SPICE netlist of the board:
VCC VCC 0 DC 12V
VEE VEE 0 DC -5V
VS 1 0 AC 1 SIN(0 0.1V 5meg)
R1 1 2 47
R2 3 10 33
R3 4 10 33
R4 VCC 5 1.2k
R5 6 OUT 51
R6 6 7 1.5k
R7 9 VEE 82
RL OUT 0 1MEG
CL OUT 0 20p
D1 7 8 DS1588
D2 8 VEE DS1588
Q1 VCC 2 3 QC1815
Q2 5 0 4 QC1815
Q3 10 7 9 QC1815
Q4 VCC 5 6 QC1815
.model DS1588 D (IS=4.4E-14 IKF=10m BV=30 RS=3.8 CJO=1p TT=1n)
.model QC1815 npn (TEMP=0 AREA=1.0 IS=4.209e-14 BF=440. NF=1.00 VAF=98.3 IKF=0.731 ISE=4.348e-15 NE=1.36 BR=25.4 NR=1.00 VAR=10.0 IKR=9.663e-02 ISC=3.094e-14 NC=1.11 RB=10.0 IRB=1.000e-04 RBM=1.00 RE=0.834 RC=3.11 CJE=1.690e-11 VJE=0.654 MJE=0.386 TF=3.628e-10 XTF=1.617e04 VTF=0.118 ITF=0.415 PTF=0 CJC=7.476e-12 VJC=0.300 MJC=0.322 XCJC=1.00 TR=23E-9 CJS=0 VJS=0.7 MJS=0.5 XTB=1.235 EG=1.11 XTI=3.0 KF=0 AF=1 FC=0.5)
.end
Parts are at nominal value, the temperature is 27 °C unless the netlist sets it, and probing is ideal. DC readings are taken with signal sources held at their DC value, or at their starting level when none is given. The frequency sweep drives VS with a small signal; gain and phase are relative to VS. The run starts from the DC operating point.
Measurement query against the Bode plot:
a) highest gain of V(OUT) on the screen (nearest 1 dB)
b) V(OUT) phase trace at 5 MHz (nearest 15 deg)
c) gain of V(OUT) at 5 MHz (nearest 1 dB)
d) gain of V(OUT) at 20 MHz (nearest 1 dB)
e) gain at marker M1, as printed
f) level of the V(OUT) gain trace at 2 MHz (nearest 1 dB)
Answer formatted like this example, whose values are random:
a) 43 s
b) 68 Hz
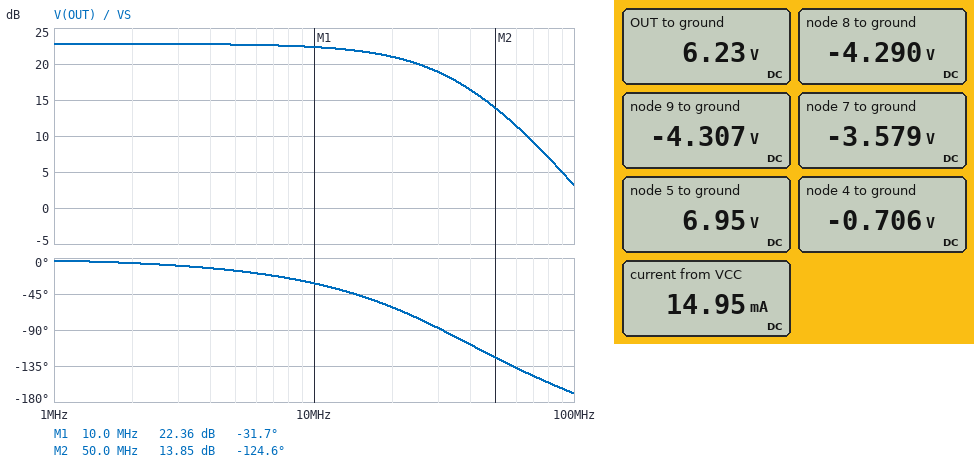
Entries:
a) 23 dB
b) -15 deg
c) 23 dB
d) 21 dB
e) 22.36 dB
f) 23 dB
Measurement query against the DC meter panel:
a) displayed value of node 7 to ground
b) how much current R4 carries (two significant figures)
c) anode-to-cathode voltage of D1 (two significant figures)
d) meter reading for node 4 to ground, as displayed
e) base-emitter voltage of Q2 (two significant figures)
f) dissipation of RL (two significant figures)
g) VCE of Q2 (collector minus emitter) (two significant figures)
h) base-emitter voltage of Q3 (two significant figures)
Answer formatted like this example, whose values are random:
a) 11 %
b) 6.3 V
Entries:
a) -3.579 V
b) 4.2 mA
c) 710 mV
d) -0.706 V
e) 710 mV
f) 39 µW
g) 7.7 V
h) 730 mV
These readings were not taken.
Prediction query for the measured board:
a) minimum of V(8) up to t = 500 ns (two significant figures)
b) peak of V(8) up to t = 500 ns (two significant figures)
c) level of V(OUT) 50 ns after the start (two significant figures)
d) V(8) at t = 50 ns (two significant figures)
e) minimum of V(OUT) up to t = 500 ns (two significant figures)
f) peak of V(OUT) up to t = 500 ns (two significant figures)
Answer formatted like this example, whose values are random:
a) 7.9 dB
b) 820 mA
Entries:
a) -4.3 V
b) -4.3 V
c) 7.5 V
d) -4.3 V
e) 4.9 V
f) 7.6 V
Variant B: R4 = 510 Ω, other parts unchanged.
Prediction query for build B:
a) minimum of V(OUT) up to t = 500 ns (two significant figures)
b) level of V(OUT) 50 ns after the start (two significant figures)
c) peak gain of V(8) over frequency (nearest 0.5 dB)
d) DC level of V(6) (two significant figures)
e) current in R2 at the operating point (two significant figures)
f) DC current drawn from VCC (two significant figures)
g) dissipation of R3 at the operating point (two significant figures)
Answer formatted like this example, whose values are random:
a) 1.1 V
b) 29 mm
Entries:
a) 8.4 V
b) 9.6 V
c) -29.5 dB
d) 9.0 V
e) 4.4 mA
f) 17 mA
g) 640 µW
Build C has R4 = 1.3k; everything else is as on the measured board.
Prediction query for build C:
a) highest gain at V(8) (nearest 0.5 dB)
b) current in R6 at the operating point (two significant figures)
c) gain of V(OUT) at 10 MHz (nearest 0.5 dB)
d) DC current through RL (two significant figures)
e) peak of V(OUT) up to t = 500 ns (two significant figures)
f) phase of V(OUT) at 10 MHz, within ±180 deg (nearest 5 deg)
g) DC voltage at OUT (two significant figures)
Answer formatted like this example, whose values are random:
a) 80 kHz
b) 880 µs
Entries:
a) -20.5 dB
b) 6.3 mA
c) 23.0 dB
d) 5.8 µA
e) 7.3 V
f) -35 deg
g) 5.8 V
